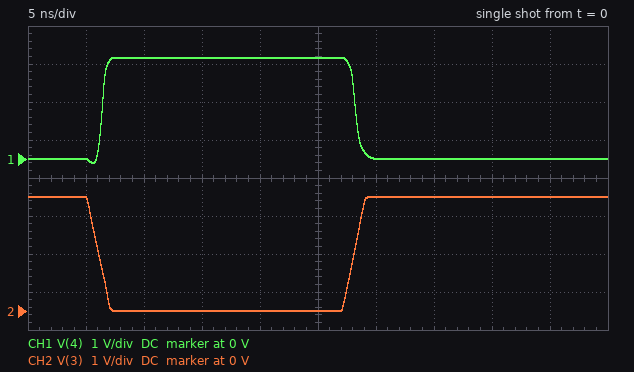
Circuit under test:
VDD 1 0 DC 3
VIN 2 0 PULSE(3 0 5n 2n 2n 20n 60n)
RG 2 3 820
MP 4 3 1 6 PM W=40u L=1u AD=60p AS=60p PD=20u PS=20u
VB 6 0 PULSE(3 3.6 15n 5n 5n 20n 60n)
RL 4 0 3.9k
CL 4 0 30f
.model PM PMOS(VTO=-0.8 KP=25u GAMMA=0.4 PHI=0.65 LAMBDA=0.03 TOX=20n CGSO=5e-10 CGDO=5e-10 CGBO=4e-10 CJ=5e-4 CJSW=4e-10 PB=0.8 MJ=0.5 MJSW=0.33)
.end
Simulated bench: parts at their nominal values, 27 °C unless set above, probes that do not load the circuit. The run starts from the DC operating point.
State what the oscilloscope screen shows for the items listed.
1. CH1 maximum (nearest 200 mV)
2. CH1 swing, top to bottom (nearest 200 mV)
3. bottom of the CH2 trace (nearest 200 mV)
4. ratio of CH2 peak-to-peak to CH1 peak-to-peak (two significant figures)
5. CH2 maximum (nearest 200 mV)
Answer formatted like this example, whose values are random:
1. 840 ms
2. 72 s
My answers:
1. 2.6 V
2. 2.8 V
3. 0 V
4. 1.1
5. 3.0 V
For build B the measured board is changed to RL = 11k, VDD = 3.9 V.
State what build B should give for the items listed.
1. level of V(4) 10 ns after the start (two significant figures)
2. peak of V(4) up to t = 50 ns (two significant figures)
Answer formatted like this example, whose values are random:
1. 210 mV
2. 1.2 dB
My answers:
1. 3.6 V
2. 3.8 V
